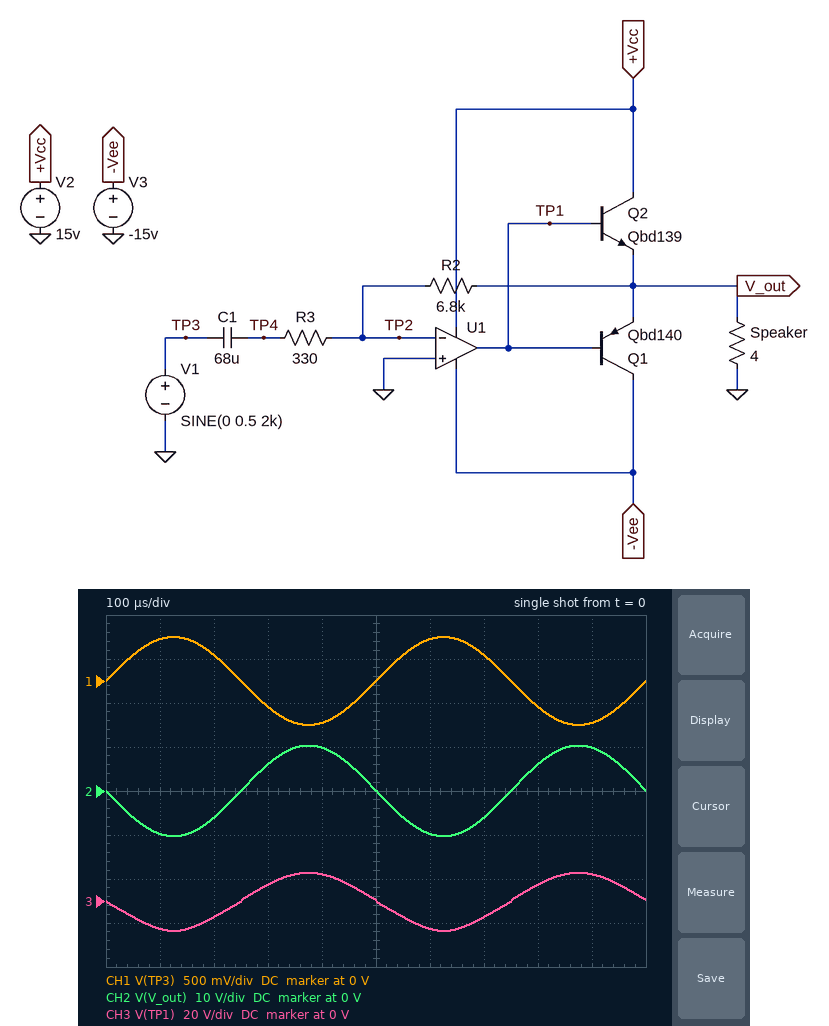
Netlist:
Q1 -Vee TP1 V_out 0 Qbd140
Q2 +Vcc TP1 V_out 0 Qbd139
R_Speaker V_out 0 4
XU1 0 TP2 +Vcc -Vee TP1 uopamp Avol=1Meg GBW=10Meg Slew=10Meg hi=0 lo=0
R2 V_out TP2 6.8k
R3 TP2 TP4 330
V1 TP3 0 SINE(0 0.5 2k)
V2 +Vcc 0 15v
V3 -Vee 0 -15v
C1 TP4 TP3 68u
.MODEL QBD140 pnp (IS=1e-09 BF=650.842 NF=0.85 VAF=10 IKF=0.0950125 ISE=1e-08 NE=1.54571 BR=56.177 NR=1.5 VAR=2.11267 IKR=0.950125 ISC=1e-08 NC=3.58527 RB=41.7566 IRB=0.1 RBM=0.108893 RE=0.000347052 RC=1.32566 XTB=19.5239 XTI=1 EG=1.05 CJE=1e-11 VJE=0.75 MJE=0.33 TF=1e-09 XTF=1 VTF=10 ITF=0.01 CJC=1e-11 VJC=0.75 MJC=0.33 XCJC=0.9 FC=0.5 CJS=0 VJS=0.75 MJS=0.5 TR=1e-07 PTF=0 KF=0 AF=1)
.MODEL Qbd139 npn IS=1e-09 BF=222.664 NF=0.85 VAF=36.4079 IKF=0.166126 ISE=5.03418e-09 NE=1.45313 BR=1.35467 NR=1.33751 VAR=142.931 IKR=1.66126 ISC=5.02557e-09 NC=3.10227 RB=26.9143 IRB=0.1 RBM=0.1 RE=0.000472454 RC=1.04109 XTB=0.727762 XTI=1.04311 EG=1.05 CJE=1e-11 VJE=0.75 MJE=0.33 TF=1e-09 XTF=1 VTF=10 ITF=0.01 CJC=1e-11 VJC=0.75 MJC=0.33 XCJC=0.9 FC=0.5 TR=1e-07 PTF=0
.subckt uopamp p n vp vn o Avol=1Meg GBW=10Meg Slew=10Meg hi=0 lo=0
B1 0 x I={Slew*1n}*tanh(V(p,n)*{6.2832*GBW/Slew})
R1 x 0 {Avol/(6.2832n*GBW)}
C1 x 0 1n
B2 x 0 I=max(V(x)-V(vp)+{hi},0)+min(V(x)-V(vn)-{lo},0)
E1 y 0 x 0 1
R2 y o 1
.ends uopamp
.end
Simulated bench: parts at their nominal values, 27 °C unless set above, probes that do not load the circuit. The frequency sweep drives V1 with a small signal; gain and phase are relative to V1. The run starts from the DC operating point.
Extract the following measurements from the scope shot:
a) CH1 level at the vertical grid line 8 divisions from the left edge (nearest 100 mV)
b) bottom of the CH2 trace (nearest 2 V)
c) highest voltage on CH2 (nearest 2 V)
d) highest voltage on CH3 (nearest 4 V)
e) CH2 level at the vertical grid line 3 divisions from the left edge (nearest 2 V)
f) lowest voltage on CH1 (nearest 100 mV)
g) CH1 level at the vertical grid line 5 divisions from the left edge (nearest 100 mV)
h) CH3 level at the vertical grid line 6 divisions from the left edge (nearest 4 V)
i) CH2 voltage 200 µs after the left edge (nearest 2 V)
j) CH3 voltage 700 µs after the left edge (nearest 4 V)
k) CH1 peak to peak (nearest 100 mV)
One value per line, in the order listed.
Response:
-300 mV
-10 V
10 V
12 V
6 V
-500 mV
0 V
-12 V
-6 V
-8 V
1.0 V
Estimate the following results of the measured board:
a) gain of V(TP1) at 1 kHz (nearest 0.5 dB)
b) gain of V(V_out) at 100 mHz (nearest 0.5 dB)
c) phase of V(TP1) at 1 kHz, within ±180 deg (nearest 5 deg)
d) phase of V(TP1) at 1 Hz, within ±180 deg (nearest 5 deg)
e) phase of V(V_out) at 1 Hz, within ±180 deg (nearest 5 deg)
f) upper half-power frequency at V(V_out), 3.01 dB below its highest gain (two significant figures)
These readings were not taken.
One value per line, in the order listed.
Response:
79.5 dB
-14.0 dB
90 deg
-140 deg
-140 deg
12 Hz
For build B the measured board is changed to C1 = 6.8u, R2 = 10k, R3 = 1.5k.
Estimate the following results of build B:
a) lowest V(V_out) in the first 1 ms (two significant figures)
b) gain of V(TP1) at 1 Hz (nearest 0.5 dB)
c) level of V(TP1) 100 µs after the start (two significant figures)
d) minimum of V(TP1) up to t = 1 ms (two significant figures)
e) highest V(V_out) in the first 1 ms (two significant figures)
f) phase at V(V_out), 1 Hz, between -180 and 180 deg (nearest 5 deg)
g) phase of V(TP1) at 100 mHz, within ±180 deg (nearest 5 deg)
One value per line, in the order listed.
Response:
-3.3 V
102.5 dB
-3.8 V
-4.0 V
3.4 V
-105 deg
-90 deg
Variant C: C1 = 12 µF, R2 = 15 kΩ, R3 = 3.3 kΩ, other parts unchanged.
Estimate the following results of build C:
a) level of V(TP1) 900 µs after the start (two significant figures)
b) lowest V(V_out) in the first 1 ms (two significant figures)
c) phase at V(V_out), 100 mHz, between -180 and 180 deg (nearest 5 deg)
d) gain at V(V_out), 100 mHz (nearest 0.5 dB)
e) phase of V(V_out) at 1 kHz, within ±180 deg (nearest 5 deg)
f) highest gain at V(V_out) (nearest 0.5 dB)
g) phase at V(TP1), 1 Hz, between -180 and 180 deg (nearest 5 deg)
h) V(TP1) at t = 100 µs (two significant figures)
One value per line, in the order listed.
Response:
2.8 V
-2.3 V
-95 deg
-22.0 dB
105 deg
2.0 dB
-125 deg
-2.7 V
